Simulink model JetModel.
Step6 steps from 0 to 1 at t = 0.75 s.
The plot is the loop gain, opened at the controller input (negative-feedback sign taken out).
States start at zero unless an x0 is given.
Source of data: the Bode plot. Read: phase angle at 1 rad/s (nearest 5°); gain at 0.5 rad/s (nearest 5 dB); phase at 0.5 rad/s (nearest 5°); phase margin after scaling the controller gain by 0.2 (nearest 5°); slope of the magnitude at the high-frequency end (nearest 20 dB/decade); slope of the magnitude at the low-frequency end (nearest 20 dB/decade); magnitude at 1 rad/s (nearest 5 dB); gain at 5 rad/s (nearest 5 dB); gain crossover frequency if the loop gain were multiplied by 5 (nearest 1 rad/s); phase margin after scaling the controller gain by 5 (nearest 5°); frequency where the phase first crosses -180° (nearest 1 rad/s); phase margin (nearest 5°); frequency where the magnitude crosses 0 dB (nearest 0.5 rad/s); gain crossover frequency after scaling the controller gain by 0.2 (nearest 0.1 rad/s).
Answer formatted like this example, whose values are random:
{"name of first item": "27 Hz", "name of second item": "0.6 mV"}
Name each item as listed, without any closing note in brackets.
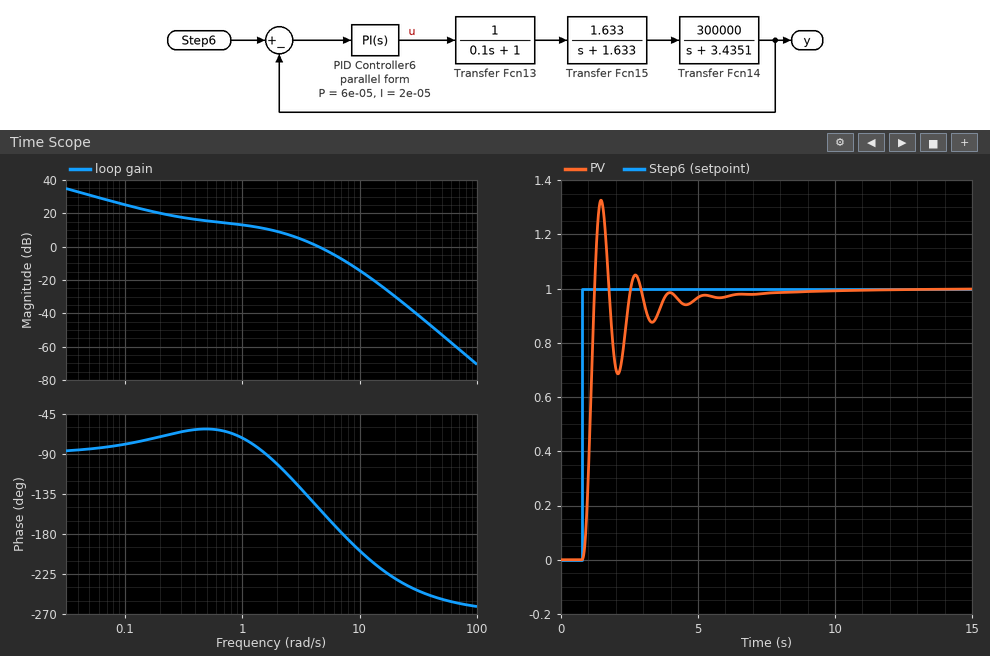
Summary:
{"phase angle at 1 rad/s": "-70°", "gain at 0.5 rad/s": "15 dB", "phase at 0.5 rad/s": "-60°", "phase margin after scaling the controller gain by 0.2": "115°", "slope of the magnitude at the high-frequency end": "-60 dB/decade", "slope of the magnitude at the low-frequency end": "-20 dB/decade", "magnitude at 1 rad/s": "15 dB", "gain at 5 rad/s": "0 dB", "gain crossover frequency if the loop gain were multiplied by 5": "10 rad/s", "phase margin after scaling the controller gain by 5": "-20°", "frequency where the phase first crosses -180°": "7 rad/s", "phase margin": "30°", "frequency where the magnitude crosses 0 dB": "4.5 rad/s", "gain crossover frequency after scaling the controller gain by 0.2": "0.8 rad/s"}
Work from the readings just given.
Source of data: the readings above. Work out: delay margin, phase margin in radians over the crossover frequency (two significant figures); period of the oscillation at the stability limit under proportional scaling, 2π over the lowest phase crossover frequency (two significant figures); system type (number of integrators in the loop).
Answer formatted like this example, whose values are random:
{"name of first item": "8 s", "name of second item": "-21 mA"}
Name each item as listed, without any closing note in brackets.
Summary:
{"delay margin, phase margin in radians over the crossover frequency": "0.12 s", "period of the oscillation at the stability limit under proportional scaling, 2π over the lowest phase crossover frequency": "0.90 s", "system type": "1"}
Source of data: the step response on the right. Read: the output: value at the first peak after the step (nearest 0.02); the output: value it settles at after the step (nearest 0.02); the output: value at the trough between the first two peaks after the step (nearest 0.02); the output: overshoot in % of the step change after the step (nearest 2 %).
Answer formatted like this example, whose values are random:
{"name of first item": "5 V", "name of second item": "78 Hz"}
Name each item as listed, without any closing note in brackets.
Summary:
{"the output: value at the first peak after the step": "1.32", "the output: value it settles at after the step": "1.00", "the output: value at the trough between the first two peaks after the step": "0.68", "the output: overshoot in % of the step change after the step": "32 %"}
